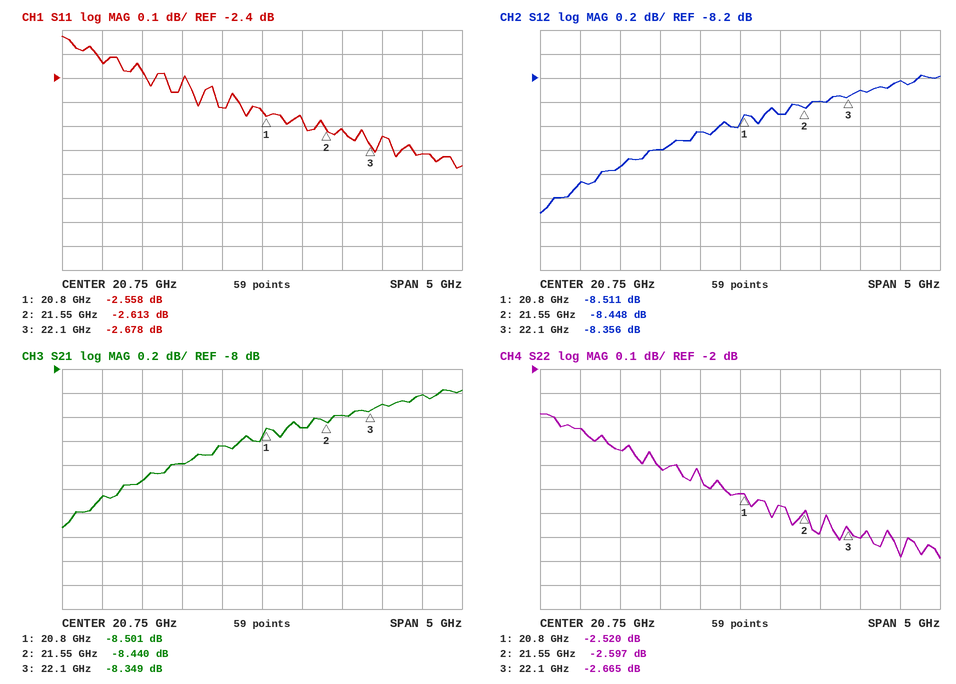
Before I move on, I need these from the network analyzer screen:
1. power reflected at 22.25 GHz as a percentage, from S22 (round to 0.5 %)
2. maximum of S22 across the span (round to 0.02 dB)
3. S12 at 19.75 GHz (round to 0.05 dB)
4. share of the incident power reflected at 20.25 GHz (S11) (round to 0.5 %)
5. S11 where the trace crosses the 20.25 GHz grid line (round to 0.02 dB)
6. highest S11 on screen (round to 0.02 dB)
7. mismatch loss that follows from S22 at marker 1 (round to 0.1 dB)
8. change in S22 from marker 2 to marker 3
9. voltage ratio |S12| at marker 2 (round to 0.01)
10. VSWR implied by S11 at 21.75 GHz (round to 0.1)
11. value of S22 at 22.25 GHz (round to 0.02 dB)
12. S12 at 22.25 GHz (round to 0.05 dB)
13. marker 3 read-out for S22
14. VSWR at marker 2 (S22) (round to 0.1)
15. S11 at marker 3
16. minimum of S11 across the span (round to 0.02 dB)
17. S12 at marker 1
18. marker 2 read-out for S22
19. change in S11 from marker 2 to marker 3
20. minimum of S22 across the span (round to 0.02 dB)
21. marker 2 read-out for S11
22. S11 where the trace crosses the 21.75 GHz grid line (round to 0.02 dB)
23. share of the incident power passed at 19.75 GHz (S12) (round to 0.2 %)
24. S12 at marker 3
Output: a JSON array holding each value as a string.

["53.5 %", "-2.18 dB", "-8.80 dB", "56.0 %", "-2.52 dB", "-2.22 dB", "3.6 dB", "-0.068 dB", "0.38", "6.7", "-2.70 dB", "-8.30 dB", "-2.665 dB", "6.7", "-2.678 dB", "-2.78 dB", "-8.511 dB", "-2.597 dB", "-0.065 dB", "-2.78 dB", "-2.613 dB", "-2.62 dB", "13.2 %", "-8.356 dB"]
